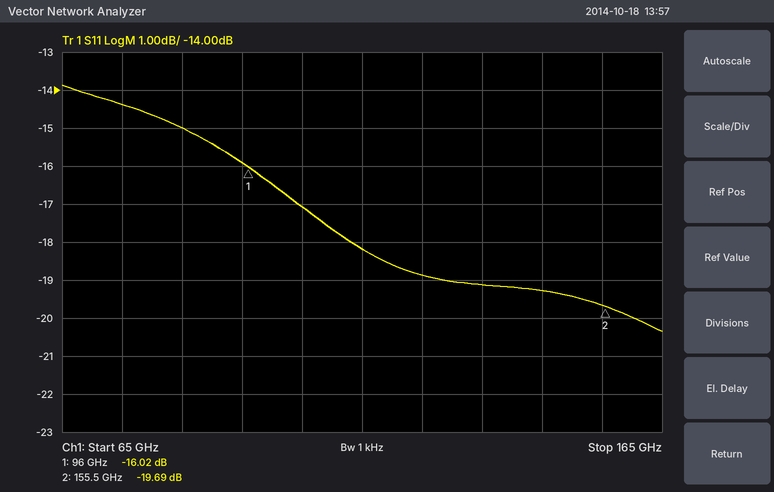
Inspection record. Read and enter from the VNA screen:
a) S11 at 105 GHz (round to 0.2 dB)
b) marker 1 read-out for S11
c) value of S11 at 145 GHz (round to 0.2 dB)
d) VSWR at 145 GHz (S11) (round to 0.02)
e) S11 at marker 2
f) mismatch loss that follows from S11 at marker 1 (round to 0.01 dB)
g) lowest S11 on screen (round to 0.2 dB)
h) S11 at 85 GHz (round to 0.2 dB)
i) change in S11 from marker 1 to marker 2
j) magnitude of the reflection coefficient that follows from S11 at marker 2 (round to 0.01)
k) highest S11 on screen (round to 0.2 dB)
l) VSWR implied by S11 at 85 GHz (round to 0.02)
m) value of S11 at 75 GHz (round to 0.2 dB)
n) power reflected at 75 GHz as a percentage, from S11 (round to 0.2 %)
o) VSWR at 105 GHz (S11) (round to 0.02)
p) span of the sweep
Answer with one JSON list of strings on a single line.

["-17.0 dB", "-16.02 dB", "-19.2 dB", "1.24", "-19.69 dB", "0.11 dB", "-20.4 dB", "-15.0 dB", "-3.67 dB", "0.10", "-13.8 dB", "1.44", "-14.4 dB", "3.6 %", "1.32", "100 GHz"]
